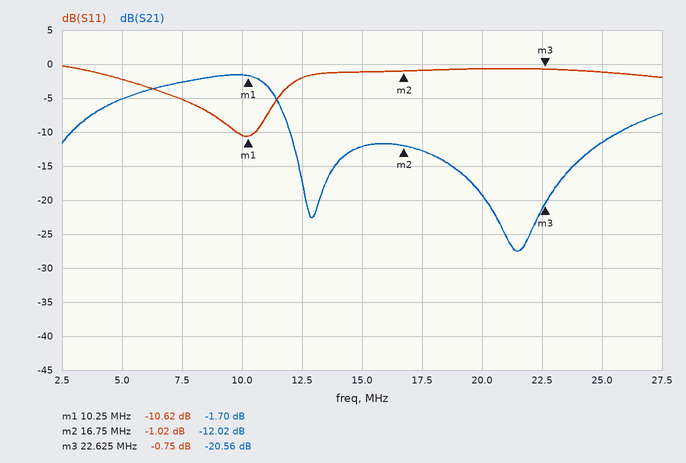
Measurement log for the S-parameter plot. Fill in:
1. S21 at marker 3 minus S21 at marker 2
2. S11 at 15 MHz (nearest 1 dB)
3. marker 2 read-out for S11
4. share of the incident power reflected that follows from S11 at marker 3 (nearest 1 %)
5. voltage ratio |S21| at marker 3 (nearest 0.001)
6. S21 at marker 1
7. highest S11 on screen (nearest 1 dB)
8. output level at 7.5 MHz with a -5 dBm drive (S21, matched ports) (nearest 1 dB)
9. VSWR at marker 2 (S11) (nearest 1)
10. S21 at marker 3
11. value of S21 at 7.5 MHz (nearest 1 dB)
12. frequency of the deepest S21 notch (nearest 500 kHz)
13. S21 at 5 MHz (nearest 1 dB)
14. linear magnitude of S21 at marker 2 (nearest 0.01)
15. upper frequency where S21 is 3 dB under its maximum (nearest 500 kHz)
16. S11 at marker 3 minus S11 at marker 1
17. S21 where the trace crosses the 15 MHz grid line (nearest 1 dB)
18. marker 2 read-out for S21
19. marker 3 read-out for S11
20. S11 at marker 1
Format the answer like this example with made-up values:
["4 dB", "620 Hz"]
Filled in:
["-8.54 dB", "-1 dB", "-1.02 dB", "84 %", "0.094", "-1.70 dB", "0 dB", "-8 dBm", "17", "-20.56 dB", "-3 dB", "21.5 MHz", "-5 dB", "0.25", "11.5 MHz", "9.87 dB", "-12 dB", "-12.02 dB", "-0.75 dB", "-10.62 dB"]
